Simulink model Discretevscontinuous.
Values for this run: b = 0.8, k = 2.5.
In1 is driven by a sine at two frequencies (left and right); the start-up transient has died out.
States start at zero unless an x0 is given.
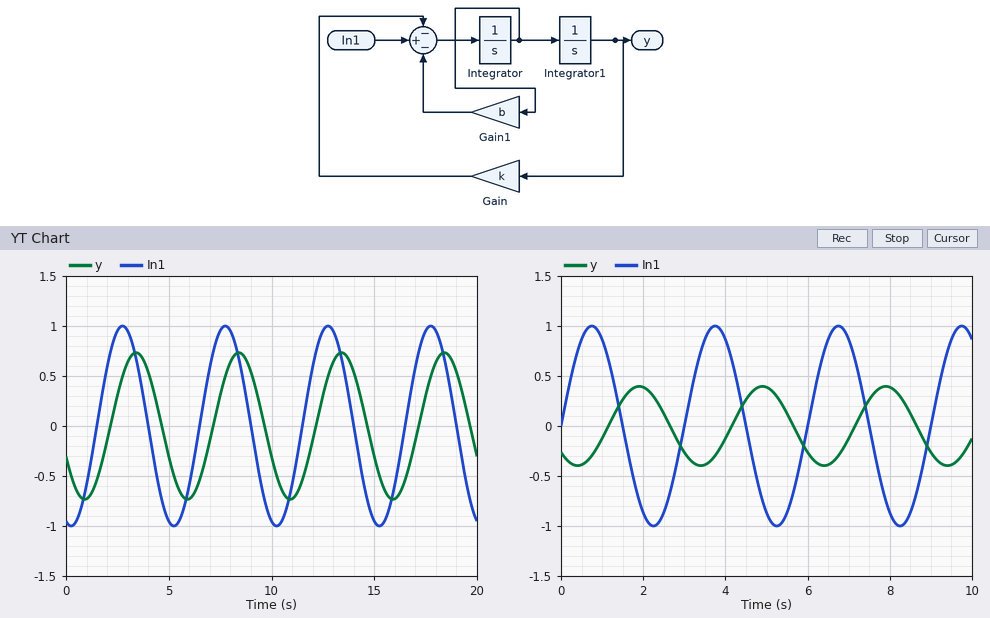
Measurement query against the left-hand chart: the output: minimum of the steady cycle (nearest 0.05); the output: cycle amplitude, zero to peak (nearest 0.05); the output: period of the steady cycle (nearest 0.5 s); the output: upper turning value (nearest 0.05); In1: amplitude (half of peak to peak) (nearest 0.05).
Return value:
-0.75
0.75
5.0 s
0.75
1.00
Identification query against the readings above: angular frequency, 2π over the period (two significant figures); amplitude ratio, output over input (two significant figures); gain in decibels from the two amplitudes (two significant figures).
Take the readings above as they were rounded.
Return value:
1.3 rad/s
0.75
-2.5 dB
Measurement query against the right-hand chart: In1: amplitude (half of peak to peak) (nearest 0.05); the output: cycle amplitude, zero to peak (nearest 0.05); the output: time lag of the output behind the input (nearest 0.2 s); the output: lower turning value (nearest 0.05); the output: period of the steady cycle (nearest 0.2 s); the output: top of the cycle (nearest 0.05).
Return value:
1.00
0.40
1.2 s
-0.40
3.0 s
0.40
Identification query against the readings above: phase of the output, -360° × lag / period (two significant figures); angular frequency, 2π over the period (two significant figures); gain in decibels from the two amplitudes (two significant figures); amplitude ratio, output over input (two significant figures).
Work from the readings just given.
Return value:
-140°
2.1 rad/s
-8.0 dB
0.40
